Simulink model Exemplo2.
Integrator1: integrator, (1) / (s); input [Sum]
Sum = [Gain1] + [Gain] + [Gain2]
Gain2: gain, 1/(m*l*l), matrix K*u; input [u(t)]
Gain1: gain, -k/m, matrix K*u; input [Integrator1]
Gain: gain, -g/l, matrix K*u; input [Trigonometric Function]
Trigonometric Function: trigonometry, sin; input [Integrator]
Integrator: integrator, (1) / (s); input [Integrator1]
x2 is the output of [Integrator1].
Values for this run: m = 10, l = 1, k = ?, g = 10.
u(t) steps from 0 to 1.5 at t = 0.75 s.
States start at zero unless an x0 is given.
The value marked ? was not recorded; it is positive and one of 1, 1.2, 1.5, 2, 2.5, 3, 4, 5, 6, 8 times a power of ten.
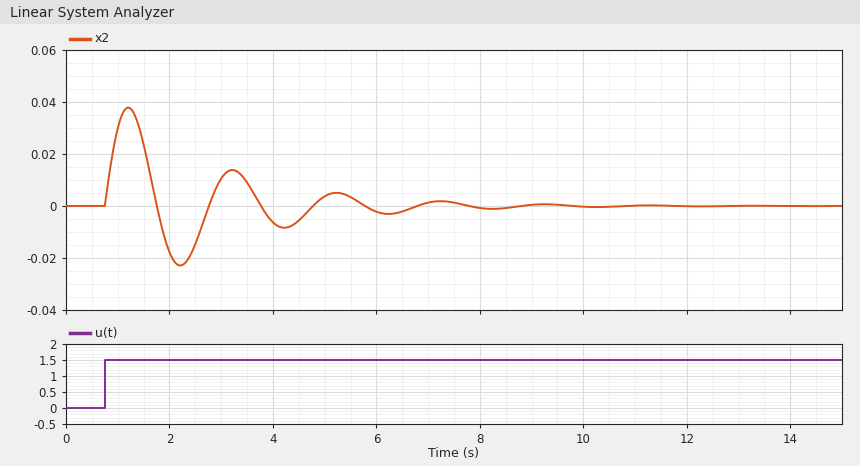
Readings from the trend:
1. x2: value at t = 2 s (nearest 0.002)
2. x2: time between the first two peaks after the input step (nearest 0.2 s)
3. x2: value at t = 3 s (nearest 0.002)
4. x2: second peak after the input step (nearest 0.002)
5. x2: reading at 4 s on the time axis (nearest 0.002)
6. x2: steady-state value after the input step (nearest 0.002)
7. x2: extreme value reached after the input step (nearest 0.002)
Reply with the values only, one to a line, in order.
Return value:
-0.018
2.0 s
0.010
0.014
-0.006
0.000
0.038
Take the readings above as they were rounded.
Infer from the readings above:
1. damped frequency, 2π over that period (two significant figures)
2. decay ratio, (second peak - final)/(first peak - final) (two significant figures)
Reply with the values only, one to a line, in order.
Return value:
3.1 rad/s
0.37
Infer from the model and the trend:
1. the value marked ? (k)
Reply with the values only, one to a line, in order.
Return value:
10
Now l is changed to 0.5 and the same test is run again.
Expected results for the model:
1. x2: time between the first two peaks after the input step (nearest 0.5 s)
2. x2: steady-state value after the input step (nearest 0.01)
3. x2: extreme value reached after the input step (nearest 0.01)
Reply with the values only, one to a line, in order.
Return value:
1.5 s
0.00
0.11
